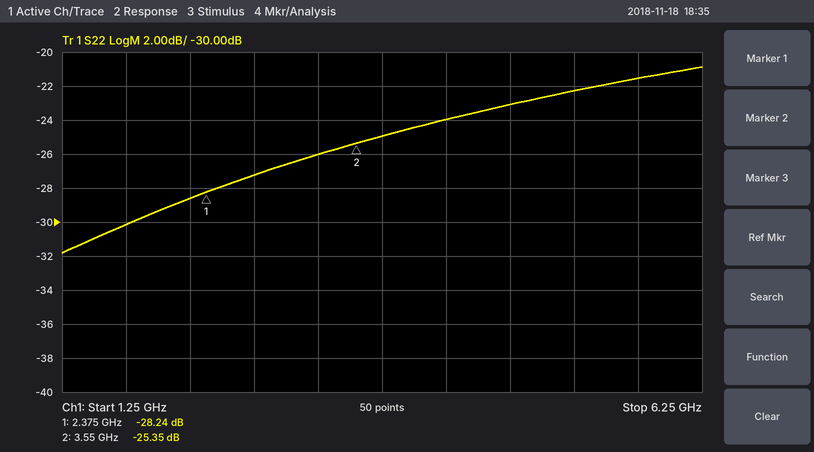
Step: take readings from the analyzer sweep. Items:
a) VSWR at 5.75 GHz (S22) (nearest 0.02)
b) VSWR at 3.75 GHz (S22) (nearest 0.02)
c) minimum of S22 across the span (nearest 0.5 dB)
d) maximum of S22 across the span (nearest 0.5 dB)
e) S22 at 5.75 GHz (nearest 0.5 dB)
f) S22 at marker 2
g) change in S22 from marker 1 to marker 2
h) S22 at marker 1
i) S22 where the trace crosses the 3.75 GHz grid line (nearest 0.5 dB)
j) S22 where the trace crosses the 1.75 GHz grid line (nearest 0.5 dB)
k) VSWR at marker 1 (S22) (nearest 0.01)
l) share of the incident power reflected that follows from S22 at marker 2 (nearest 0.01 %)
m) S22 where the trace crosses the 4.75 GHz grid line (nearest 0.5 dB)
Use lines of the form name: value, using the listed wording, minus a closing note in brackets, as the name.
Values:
VSWR at 5.75 GHz (S22): 1.18
VSWR at 3.75 GHz (S22): 1.12
minimum of S22 across the span: -32.0 dB
maximum of S22 across the span: -21.0 dB
S22 at 5.75 GHz: -21.5 dB
S22 at marker 2: -25.35 dB
change in S22 from marker 1 to marker 2: 2.89 dB
S22 at marker 1: -28.24 dB
S22 where the trace crosses the 3.75 GHz grid line: -25.0 dB
S22 where the trace crosses the 1.75 GHz grid line: -30.0 dB
VSWR at marker 1 (S22): 1.08
share of the incident power reflected that follows from S22 at marker 2: 0.29 %
S22 where the trace crosses the 4.75 GHz grid line: -23.0 dB
